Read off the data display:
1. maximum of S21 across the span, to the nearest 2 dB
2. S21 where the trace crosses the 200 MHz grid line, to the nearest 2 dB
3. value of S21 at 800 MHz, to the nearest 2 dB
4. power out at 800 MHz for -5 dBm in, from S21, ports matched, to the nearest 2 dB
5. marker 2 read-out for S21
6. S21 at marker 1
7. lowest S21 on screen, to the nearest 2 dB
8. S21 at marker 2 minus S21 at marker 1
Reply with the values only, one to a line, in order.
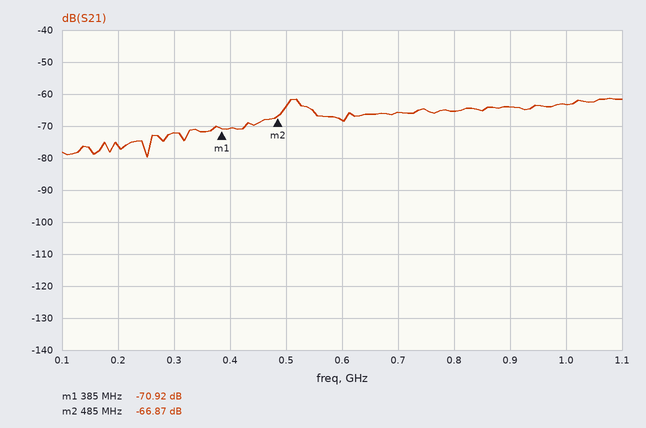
-62 dB
-76 dB
-66 dB
-70 dBm
-66.87 dB
-70.92 dB
-80 dB
4.05 dB
